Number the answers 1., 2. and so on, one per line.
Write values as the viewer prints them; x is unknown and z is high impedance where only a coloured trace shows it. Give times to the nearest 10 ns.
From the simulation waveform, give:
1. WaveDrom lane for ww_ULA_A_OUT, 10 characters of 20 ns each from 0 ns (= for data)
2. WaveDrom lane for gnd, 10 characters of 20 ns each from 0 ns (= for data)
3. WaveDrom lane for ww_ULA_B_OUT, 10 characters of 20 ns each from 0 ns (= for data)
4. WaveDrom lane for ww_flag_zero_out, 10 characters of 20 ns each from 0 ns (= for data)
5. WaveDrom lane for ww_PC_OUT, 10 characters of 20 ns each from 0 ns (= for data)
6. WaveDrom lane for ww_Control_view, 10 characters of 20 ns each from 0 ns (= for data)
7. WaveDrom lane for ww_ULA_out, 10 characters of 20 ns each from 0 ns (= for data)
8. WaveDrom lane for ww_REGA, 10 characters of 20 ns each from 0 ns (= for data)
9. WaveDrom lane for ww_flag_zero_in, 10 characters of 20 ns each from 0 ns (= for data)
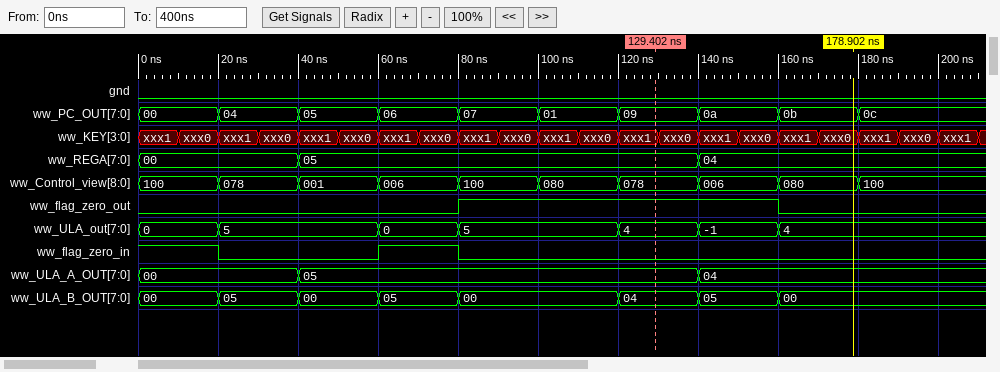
1. {name: 'ww_ULA_A_OUT', wave: '=.=....=..', data: '00 05 04'}
2. {name: 'gnd', wave: '0.........'}
3. {name: 'ww_ULA_B_OUT', wave: '=====.===.', data: '00 05 00 05 00 04 05 00'}
4. {name: 'ww_flag_zero_out', wave: '0...1...0.'}
5. {name: 'ww_PC_OUT', wave: '==========', data: '00 04 05 06 07 01 09 0a 0b 0c'}
6. {name: 'ww_Control_view', wave: '==========', data: '100 078 001 006 100 080 078 006 080 100'}
7. {name: 'ww_ULA_out', wave: '==.==.===.', data: '0 5 0 5 4 -1 4'}
8. {name: 'ww_REGA', wave: '=.=....=..', data: '00 05 04'}
9. {name: 'ww_flag_zero_in', wave: '10.10.....'}
